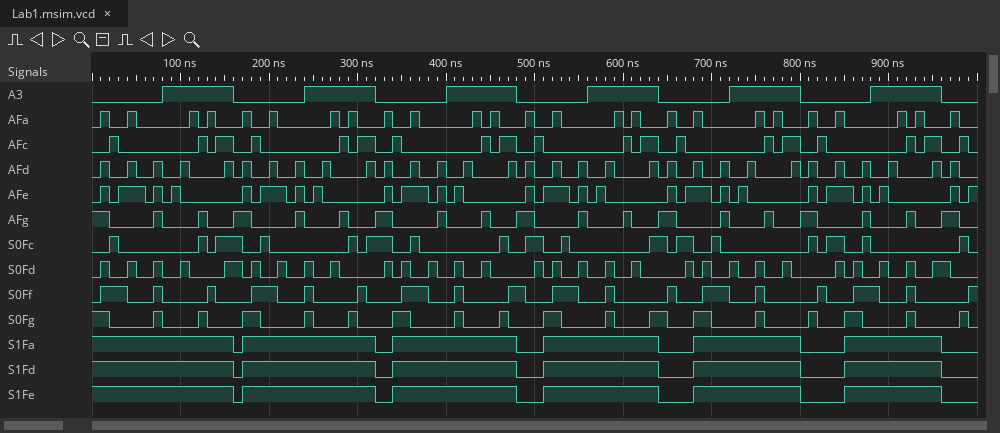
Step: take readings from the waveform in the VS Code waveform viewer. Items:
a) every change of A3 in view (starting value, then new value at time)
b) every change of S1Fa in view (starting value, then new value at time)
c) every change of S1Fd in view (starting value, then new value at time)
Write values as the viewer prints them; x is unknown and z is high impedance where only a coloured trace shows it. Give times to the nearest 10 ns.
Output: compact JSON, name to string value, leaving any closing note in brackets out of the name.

{"every change of A3 in view": "0, 1 at 80 ns, 0 at 160 ns, 1 at 240 ns, 0 at 320 ns, 1 at 400 ns, 0 at 480 ns, 1 at 560 ns, 0 at 640 ns, 1 at 720 ns, 0 at 800 ns, 1 at 880 ns, 0 at 960 ns", "every change of S1Fa in view": "1, 0 at 160 ns, 1 at 170 ns, 0 at 320 ns, 1 at 340 ns, 0 at 480 ns, 1 at 510 ns, 0 at 640 ns, 1 at 680 ns, 0 at 800 ns, 1 at 850 ns, 0 at 960 ns", "every change of S1Fd in view": "1, 0 at 160 ns, 1 at 170 ns, 0 at 320 ns, 1 at 340 ns, 0 at 480 ns, 1 at 510 ns, 0 at 640 ns, 1 at 680 ns, 0 at 800 ns, 1 at 850 ns, 0 at 960 ns"}
